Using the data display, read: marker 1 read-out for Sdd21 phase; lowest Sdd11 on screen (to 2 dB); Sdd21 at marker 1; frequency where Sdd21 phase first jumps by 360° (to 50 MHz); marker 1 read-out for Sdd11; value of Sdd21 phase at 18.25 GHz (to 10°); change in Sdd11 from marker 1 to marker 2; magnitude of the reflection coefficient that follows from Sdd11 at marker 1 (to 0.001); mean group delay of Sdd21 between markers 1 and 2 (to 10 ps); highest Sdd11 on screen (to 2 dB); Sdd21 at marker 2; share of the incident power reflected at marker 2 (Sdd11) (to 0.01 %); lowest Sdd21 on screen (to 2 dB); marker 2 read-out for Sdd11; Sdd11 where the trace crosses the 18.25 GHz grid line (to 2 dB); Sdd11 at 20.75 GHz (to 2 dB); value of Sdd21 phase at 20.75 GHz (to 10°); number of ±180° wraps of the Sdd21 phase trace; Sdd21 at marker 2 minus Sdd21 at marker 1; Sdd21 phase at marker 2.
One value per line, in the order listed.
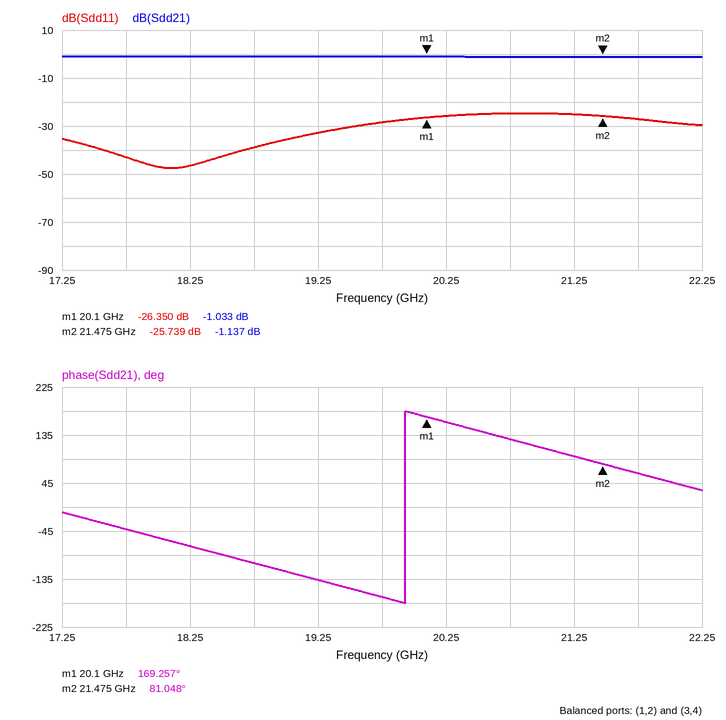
169.257°
-48 dB
-1.033 dB
19.95 GHz
-26.350 dB
-70°
0.611 dB
0.048
180 ps
-24 dB
-1.137 dB
0.27 %
-2 dB
-25.739 dB
-46 dB
-24 dB
130°
1
-0.104 dB
81.048°
